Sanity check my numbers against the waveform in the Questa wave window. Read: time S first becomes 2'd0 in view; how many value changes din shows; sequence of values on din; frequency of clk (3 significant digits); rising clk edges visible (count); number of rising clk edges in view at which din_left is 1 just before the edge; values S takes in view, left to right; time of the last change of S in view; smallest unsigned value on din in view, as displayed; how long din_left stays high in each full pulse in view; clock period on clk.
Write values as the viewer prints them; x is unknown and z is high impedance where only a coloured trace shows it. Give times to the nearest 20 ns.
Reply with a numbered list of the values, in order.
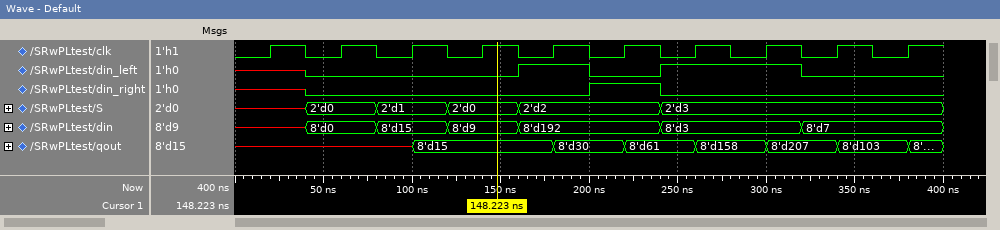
1. 40 ns
2. 6
3. x, 8'd0, 8'd15, 8'd9, 8'd192, 8'd3, 8'd7
4. 25.0 MHz
5. 10
6. 3
7. x, 2'd0, 2'd1, 2'd0, 2'd2, 2'd3
8. 240 ns
9. 8'd0
10. 40 ns, 80 ns
11. 40 ns
